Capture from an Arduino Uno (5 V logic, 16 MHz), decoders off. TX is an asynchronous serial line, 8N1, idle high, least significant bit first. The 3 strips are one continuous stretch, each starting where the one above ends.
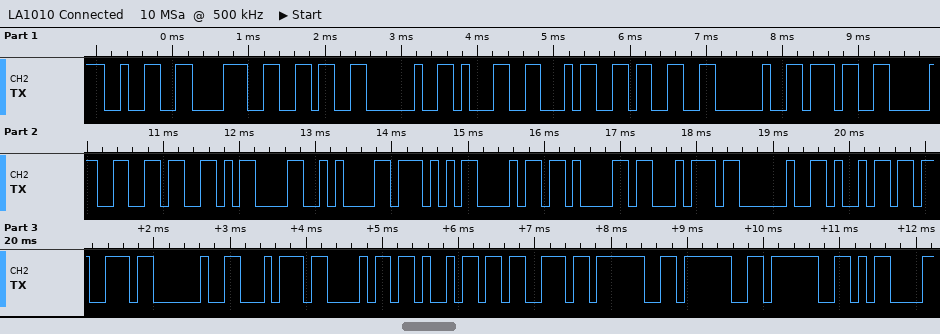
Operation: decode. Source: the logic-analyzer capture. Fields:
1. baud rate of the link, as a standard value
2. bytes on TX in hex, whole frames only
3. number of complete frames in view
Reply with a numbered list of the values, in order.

1. 9600 baud
2. 32 38 36 20 31 34 33 20 37 30 36 0D 0A 57 68 61 74 20 69 73 20 74 68 69 73 3F 3F 3F 0D
3. 29
